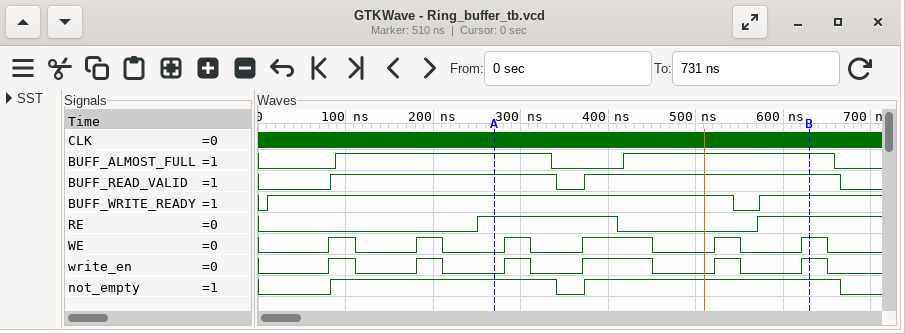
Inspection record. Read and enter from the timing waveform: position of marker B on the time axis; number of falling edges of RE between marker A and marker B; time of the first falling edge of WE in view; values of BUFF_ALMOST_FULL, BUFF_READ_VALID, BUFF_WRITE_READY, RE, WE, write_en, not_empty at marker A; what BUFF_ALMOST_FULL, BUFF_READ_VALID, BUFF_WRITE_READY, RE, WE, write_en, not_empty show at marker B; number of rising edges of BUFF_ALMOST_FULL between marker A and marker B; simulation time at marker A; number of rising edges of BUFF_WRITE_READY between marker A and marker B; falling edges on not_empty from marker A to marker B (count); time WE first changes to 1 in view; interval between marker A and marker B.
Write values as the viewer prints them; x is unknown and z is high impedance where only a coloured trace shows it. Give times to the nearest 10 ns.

630 ns
1
110 ns
BUFF_ALMOST_FULL=1, BUFF_READ_VALID=1, BUFF_WRITE_READY=1, RE=1, WE=0, write_en=0, not_empty=1
BUFF_ALMOST_FULL=1, BUFF_READ_VALID=1, BUFF_WRITE_READY=1, RE=1, WE=1, write_en=1, not_empty=1
1
270 ns
1
1
80 ns
360 ns
